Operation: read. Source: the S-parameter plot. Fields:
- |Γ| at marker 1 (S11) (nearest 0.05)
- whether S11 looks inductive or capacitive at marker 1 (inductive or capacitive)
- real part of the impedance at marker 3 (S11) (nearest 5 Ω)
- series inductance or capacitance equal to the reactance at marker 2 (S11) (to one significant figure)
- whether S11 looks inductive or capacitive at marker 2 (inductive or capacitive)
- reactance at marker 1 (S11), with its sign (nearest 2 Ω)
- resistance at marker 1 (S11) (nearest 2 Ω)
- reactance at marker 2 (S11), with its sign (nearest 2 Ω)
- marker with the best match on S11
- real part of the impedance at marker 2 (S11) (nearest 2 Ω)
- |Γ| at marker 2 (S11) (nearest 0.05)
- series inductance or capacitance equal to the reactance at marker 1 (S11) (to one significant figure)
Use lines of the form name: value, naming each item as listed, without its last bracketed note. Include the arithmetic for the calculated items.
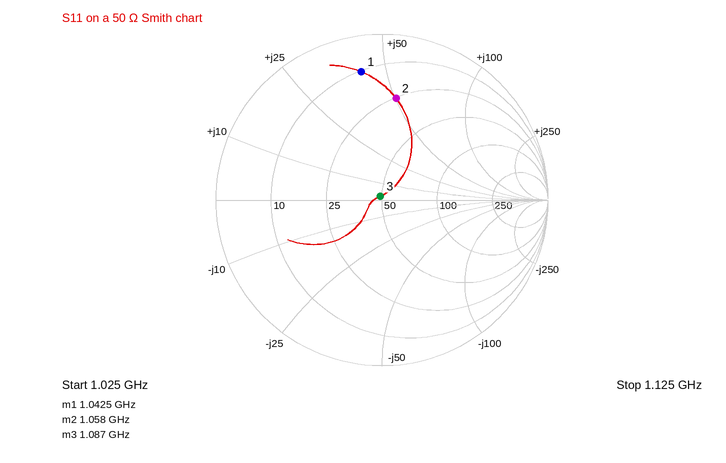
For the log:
|Γ| at marker 1 (S11): 0.80
whether S11 looks inductive or capacitive at marker 1: inductive
real part of the impedance at marker 3 (S11): 50 Ω
series inductance or capacitance equal to the reactance at marker 2 (S11): L = 50 Ω/(2π × 1.058 GHz) ≈ 8 nH
whether S11 looks inductive or capacitive at marker 2: inductive
reactance at marker 1 (S11), with its sign: +42 Ω
resistance at marker 1 (S11): 10 Ω
reactance at marker 2 (S11), with its sign: +50 Ω
marker with the best match on S11: marker 3
real part of the impedance at marker 2 (S11): 26 Ω
|Γ| at marker 2 (S11): 0.60
series inductance or capacitance equal to the reactance at marker 1 (S11): L = 42 Ω/(2π × 1.0425 GHz) ≈ 6 nH
